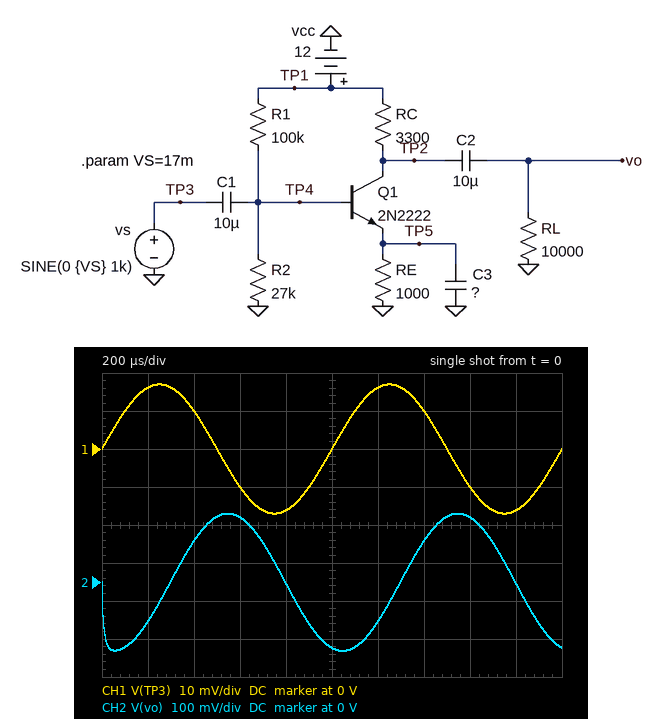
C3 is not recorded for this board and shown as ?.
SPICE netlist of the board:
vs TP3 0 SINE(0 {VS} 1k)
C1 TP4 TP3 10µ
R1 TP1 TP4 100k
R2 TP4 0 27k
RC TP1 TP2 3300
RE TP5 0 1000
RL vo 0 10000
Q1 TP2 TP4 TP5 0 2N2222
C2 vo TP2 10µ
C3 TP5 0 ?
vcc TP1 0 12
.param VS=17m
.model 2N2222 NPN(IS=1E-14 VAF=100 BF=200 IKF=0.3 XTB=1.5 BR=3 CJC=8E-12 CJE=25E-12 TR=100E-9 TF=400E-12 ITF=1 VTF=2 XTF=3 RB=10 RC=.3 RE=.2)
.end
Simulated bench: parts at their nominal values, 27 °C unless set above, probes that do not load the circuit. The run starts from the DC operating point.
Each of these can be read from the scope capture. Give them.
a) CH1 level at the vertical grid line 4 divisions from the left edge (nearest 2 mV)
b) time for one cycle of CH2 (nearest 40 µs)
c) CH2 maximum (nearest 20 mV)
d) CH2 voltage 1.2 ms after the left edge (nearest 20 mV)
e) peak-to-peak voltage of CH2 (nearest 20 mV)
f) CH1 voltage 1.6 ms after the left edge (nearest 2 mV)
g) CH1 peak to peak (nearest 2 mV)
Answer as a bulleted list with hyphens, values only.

- -16 mV
- 1.00 ms
- 180 mV
- -100 mV
- 360 mV
- -10 mV
- 34 mV
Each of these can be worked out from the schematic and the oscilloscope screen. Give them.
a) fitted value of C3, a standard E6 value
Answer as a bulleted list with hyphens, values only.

- 680 nF
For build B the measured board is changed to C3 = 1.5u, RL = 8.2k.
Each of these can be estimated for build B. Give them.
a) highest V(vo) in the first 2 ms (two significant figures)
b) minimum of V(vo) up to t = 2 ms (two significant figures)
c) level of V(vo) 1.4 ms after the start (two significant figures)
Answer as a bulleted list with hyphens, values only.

- 370 mV
- -370 mV
- 230 mV
